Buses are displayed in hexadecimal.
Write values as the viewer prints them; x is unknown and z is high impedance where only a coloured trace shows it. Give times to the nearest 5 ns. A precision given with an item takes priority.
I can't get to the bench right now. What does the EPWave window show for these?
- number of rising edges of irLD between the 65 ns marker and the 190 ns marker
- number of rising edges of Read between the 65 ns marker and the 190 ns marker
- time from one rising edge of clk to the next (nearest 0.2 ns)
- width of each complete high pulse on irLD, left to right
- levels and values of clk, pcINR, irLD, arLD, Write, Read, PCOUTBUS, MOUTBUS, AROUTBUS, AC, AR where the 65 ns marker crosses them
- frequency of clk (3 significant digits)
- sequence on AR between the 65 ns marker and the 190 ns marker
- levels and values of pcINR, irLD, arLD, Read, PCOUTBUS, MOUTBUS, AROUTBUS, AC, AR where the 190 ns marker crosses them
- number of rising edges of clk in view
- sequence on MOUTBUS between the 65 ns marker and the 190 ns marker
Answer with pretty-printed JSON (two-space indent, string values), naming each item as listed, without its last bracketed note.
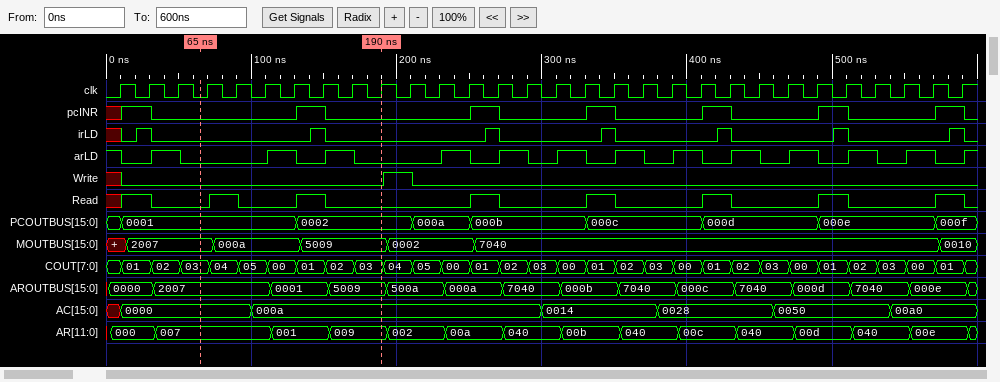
{
  "number of rising edges of irLD between the 65 ns marker and the 190 ns marker": "1",
  "number of rising edges of Read between the 65 ns marker and the 190 ns marker": "2",
  "time from one rising edge of clk to the next": "20 ns",
  "width of each complete high pulse on irLD, left to right": "10 ns, 10 ns, 10 ns, 10 ns, 10 ns, 10 ns, 10 ns",
  "levels and values of clk, pcINR, irLD, arLD, Write, Read, PCOUTBUS, MOUTBUS, AROUTBUS, AC, AR where the 65 ns marker crosses them": "clk=0, pcINR=0, irLD=0, arLD=0, Write=0, Read=0, PCOUTBUS=0001, MOUTBUS=2007, AROUTBUS=2007, AC=0000, AR=007",
  "frequency of clk": "50.0 MHz",
  "sequence on AR between the 65 ns marker and the 190 ns marker": "007, 001, 009",
  "levels and values of pcINR, irLD, arLD, Read, PCOUTBUS, MOUTBUS, AROUTBUS, AC, AR where the 190 ns marker crosses them": "pcINR=0, irLD=0, arLD=0, Read=0, PCOUTBUS=0002, MOUTBUS=5009, AROUTBUS=5009, AC=000a, AR=009",
  "number of rising edges of clk in view": "30",
  "sequence on MOUTBUS between the 65 ns marker and the 190 ns marker": "2007, 000a, 5009"
}
